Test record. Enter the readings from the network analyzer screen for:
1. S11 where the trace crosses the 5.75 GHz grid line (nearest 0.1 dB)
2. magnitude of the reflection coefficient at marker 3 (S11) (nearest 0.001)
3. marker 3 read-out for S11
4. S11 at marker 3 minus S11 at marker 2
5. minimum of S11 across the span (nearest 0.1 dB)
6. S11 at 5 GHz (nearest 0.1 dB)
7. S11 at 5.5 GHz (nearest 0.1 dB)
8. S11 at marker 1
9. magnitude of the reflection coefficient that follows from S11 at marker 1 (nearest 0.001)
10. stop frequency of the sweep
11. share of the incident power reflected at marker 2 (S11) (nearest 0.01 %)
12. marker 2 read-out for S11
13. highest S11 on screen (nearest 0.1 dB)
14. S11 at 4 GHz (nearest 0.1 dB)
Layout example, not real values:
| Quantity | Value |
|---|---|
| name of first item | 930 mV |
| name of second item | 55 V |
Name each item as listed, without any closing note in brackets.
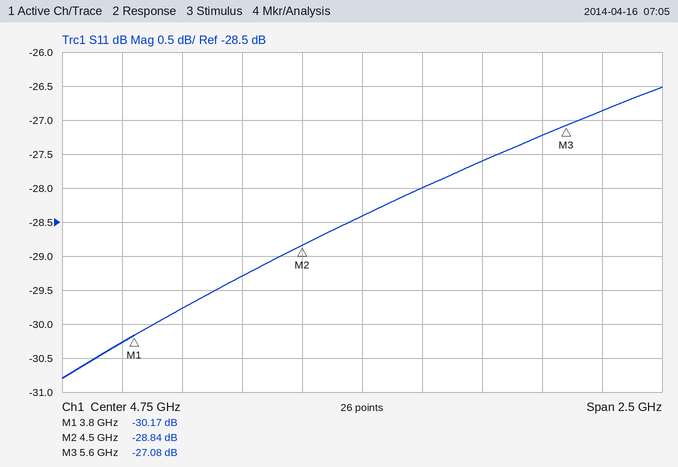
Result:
| Quantity | Value |
|---|---|
| S11 where the trace crosses the 5.75 GHz grid line | -26.9 dB |
| magnitude of the reflection coefficient at marker 3 (S11) | 0.044 |
| marker 3 read-out for S11 | -27.08 dB |
| S11 at marker 3 minus S11 at marker 2 | 1.76 dB |
| minimum of S11 across the span | -30.8 dB |
| S11 at 5 GHz | -28.0 dB |
| S11 at 5.5 GHz | -27.2 dB |
| S11 at marker 1 | -30.17 dB |
| magnitude of the reflection coefficient that follows from S11 at marker 1 | 0.031 |
| stop frequency of the sweep | 6 GHz |
| share of the incident power reflected at marker 2 (S11) | 0.13 % |
| marker 2 read-out for S11 | -28.84 dB |
| highest S11 on screen | -26.5 dB |
| S11 at 4 GHz | -29.8 dB |
